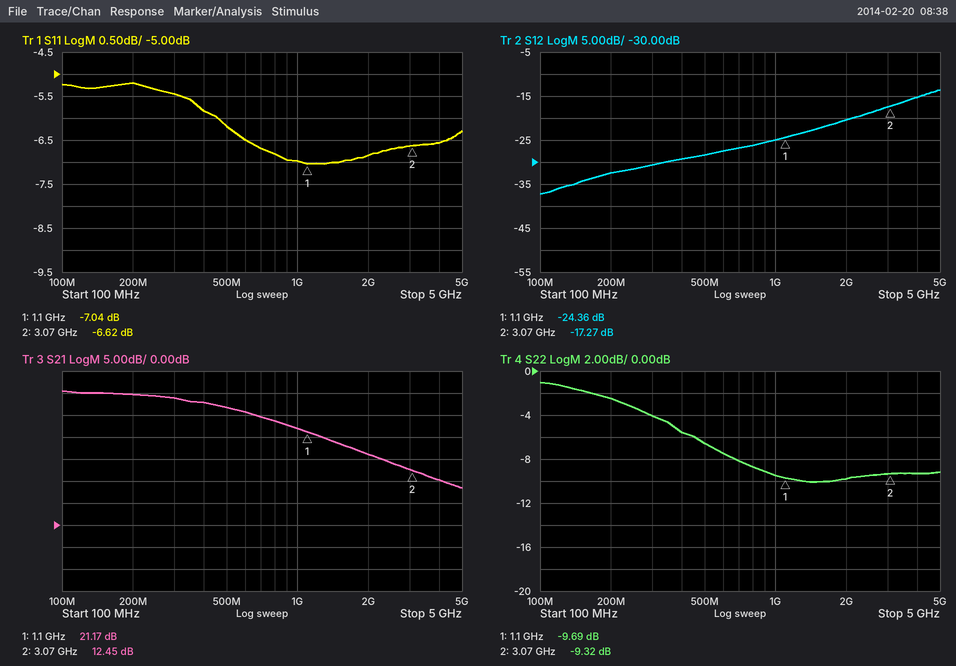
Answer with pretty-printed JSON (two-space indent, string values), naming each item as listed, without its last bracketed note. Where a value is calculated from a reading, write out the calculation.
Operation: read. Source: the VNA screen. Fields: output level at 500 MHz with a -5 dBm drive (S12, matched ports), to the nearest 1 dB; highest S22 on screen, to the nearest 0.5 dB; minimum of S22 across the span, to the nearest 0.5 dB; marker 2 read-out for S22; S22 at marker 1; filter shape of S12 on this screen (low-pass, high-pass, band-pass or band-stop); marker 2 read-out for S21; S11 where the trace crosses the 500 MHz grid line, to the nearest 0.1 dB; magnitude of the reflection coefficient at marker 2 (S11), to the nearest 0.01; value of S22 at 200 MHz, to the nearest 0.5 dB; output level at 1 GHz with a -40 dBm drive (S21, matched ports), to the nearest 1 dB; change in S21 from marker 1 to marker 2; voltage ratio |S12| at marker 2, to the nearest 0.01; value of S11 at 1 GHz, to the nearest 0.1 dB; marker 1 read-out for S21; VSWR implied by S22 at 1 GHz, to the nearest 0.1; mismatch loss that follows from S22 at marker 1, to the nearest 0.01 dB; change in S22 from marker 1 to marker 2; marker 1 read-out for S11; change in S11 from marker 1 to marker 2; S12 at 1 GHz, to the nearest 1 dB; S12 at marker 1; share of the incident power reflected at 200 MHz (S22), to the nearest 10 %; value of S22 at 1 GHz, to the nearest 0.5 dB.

{
  "output level at 500 MHz with a -5 dBm drive (S12, matched ports), to the nearest 1 dB": "-5 dBm + (-28 dB) = -33 dBm",
  "highest S22 on screen, to the nearest 0.5 dB": "-1.0 dB",
  "minimum of S22 across the span, to the nearest 0.5 dB": "-10.0 dB",
  "marker 2 read-out for S22": "-9.32 dB",
  "S22 at marker 1": "-9.69 dB",
  "filter shape of S12 on this screen": "high-pass",
  "marker 2 read-out for S21": "12.45 dB",
  "S11 where the trace crosses the 500 MHz grid line, to the nearest 0.1 dB": "-6.2 dB",
  "magnitude of the reflection coefficient at marker 2 (S11), to the nearest 0.01": "10^(-6.62/20) ≈ 0.47",
  "value of S22 at 200 MHz, to the nearest 0.5 dB": "-2.5 dB",
  "output level at 1 GHz with a -40 dBm drive (S21, matched ports), to the nearest 1 dB": "-40 dBm + (22 dB) = -18 dBm",
  "change in S21 from marker 1 to marker 2": "12.45 − (21.17) = -8.72 dB",
  "voltage ratio |S12| at marker 2, to the nearest 0.01": "10^(-17.27/20) ≈ 0.14",
  "value of S11 at 1 GHz, to the nearest 0.1 dB": "-7.0 dB",
  "marker 1 read-out for S21": "21.17 dB",
  "VSWR implied by S22 at 1 GHz, to the nearest 0.1": "|Γ| = 10^(-9.5/20) = 0.3350; VSWR = (1 + 0.3350)/(1 − 0.3350) ≈ 2.0",
  "mismatch loss that follows from S22 at marker 1, to the nearest 0.01 dB": "−10 log10(1 − 10^(-9.69/10)) ≈ 0.49 dB",
  "change in S22 from marker 1 to marker 2": "-9.32 − (-9.69) = 0.37 dB",
  "marker 1 read-out for S11": "-7.04 dB",
  "change in S11 from marker 1 to marker 2": "-6.62 − (-7.04) = 0.42 dB",
  "S12 at 1 GHz, to the nearest 1 dB": "-25 dB",
  "S12 at marker 1": "-24.36 dB",
  "share of the incident power reflected at 200 MHz (S22), to the nearest 10 %": "10^(-2.5/10) ≈ 56.2 %, so 60 % to the nearest 10 %",
  "value of S22 at 1 GHz, to the nearest 0.5 dB": "-9.5 dB"
}
